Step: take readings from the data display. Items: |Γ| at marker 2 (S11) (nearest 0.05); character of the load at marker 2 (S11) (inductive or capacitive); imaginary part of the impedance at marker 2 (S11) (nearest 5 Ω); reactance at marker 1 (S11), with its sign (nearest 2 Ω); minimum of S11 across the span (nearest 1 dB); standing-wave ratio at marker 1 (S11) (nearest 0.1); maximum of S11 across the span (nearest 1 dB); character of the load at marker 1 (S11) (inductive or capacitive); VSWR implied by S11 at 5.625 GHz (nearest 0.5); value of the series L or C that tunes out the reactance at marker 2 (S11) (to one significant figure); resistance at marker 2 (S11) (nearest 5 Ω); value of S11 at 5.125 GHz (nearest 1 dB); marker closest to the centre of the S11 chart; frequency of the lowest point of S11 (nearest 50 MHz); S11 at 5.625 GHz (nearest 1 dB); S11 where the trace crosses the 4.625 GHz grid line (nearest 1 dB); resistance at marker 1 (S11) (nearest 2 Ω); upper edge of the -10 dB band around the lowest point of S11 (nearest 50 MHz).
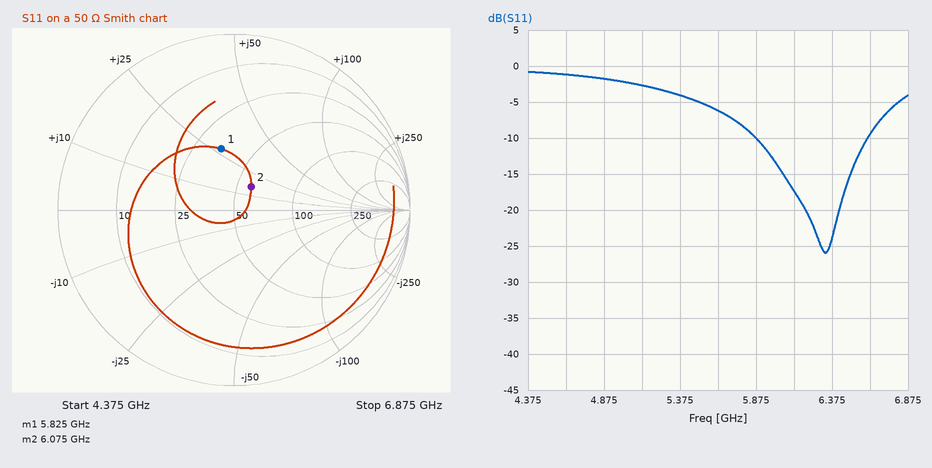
0.15
inductive
+15 Ω
+28 Ω
-26 dB
2.1
-1 dB
inductive
3.0
2 pF
60 Ω
-3 dB
marker 2
6.35 GHz
-6 dB
-1 dB
34 Ω
6.60 GHz
